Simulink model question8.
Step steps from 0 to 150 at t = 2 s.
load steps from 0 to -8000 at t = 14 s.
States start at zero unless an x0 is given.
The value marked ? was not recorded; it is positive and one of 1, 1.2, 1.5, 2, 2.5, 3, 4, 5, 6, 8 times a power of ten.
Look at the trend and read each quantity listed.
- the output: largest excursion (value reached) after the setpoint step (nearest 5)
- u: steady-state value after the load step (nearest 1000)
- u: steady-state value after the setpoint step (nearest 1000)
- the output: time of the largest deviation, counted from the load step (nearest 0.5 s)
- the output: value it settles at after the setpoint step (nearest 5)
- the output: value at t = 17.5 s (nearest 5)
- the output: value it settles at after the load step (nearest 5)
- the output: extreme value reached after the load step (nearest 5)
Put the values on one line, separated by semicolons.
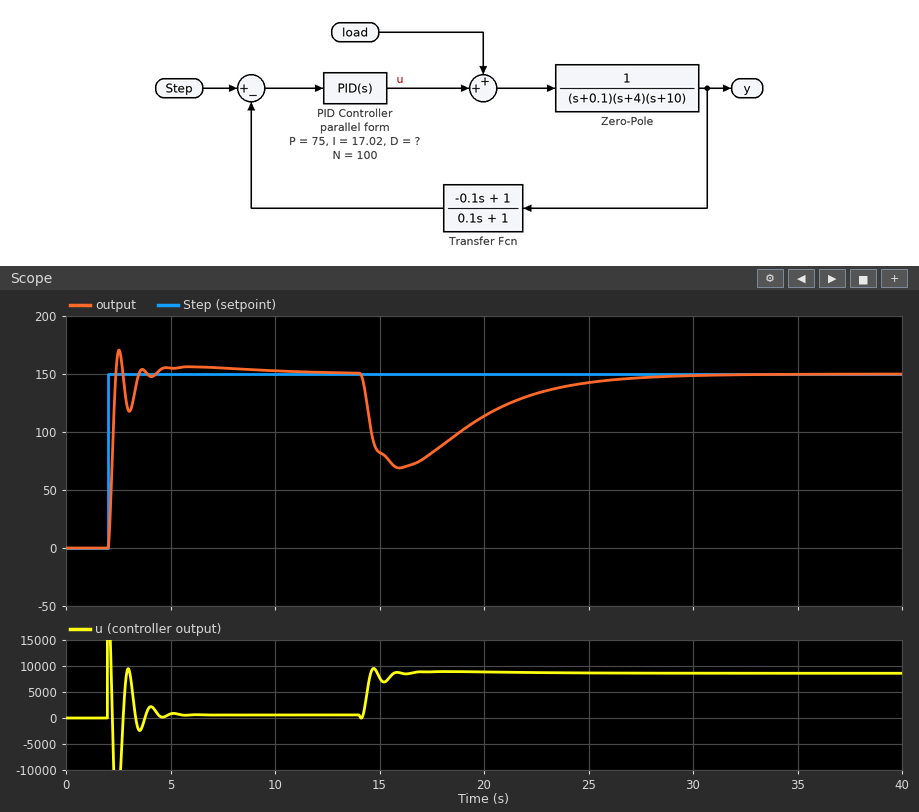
170; 9000; 1000; 2.0 s; 150; 80; 150; 70
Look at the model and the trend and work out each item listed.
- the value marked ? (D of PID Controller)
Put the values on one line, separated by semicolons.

50
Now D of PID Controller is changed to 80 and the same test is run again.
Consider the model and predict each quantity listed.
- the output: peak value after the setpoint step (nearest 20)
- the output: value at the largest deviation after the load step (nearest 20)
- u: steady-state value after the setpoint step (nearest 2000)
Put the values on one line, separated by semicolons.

220; 80; 0
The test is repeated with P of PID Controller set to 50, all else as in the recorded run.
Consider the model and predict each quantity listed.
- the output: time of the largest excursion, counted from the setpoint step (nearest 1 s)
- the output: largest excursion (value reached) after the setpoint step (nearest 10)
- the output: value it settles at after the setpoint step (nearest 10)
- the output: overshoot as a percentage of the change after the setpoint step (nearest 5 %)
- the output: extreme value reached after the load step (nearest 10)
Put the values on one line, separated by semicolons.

5 s; 160; 150; 10 %; 50
